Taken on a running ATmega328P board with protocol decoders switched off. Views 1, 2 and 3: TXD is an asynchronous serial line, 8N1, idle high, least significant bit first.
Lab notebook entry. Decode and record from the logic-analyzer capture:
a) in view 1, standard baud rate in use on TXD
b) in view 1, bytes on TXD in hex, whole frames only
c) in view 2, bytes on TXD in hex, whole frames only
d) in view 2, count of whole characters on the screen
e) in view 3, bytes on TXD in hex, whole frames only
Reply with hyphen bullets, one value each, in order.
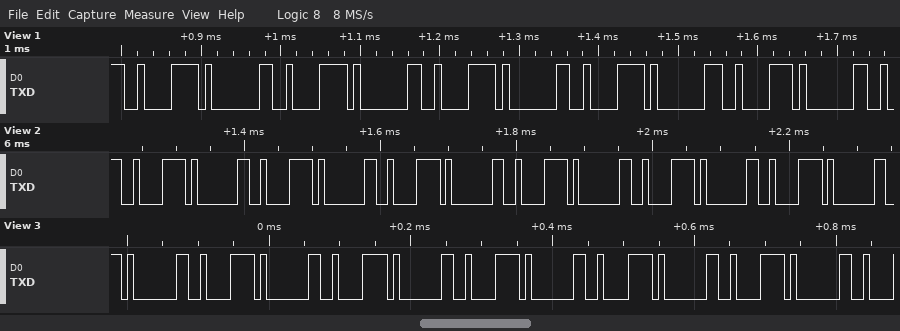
- 115200 baud
- C2 01 C2 01 C2 01 C2 01 C2 01
- C2 01 C2 01 C2 01 C2 01 C2 01 C2 01
- 12
- 01 C2 01 C2 01 C2 01 C2 01 C2 01
